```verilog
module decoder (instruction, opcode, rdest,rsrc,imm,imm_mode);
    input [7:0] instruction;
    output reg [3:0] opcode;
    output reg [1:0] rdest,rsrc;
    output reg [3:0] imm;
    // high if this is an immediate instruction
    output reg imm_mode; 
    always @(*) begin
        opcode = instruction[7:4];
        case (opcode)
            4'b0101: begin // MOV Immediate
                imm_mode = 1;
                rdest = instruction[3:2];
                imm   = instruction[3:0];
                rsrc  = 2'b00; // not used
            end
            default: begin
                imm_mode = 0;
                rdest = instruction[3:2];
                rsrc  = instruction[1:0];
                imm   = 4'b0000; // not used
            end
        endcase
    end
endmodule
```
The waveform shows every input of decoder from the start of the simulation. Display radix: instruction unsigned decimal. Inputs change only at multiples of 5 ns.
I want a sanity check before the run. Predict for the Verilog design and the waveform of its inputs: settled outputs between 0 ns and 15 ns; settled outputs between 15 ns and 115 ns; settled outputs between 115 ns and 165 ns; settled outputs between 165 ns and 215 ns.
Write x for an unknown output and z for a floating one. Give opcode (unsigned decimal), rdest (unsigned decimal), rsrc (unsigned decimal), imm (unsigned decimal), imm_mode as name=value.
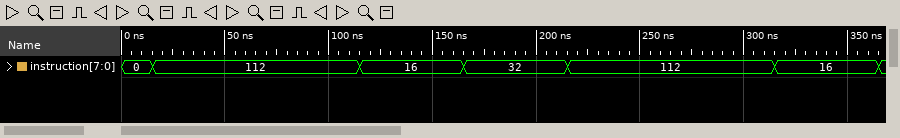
opcode=0, rdest=0, rsrc=0, imm=0, imm_mode=0
opcode=7, rdest=0, rsrc=0, imm=0, imm_mode=0
opcode=1, rdest=0, rsrc=0, imm=0, imm_mode=0
opcode=2, rdest=0, rsrc=0, imm=0, imm_mode=0
